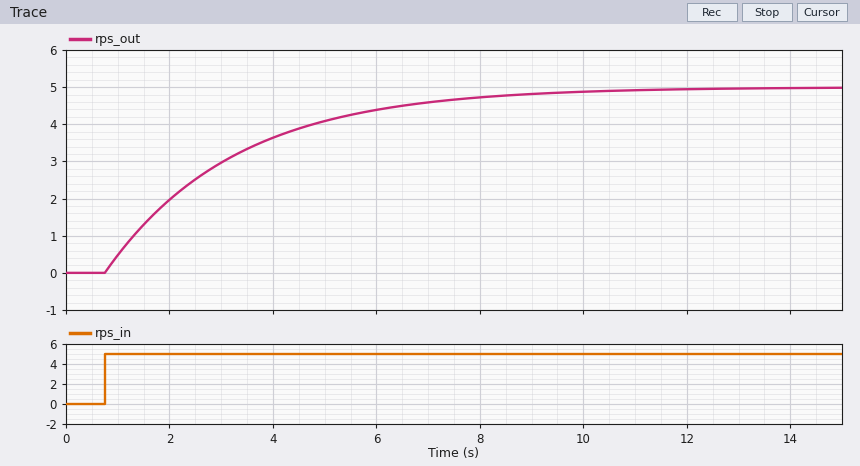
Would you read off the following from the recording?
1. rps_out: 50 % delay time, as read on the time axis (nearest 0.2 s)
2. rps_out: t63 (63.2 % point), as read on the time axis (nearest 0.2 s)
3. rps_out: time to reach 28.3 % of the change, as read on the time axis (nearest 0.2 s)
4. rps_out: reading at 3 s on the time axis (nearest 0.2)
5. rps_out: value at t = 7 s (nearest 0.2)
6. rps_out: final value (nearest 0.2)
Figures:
2.4 s
3.2 s
1.6 s
3.0
4.6
5.0
